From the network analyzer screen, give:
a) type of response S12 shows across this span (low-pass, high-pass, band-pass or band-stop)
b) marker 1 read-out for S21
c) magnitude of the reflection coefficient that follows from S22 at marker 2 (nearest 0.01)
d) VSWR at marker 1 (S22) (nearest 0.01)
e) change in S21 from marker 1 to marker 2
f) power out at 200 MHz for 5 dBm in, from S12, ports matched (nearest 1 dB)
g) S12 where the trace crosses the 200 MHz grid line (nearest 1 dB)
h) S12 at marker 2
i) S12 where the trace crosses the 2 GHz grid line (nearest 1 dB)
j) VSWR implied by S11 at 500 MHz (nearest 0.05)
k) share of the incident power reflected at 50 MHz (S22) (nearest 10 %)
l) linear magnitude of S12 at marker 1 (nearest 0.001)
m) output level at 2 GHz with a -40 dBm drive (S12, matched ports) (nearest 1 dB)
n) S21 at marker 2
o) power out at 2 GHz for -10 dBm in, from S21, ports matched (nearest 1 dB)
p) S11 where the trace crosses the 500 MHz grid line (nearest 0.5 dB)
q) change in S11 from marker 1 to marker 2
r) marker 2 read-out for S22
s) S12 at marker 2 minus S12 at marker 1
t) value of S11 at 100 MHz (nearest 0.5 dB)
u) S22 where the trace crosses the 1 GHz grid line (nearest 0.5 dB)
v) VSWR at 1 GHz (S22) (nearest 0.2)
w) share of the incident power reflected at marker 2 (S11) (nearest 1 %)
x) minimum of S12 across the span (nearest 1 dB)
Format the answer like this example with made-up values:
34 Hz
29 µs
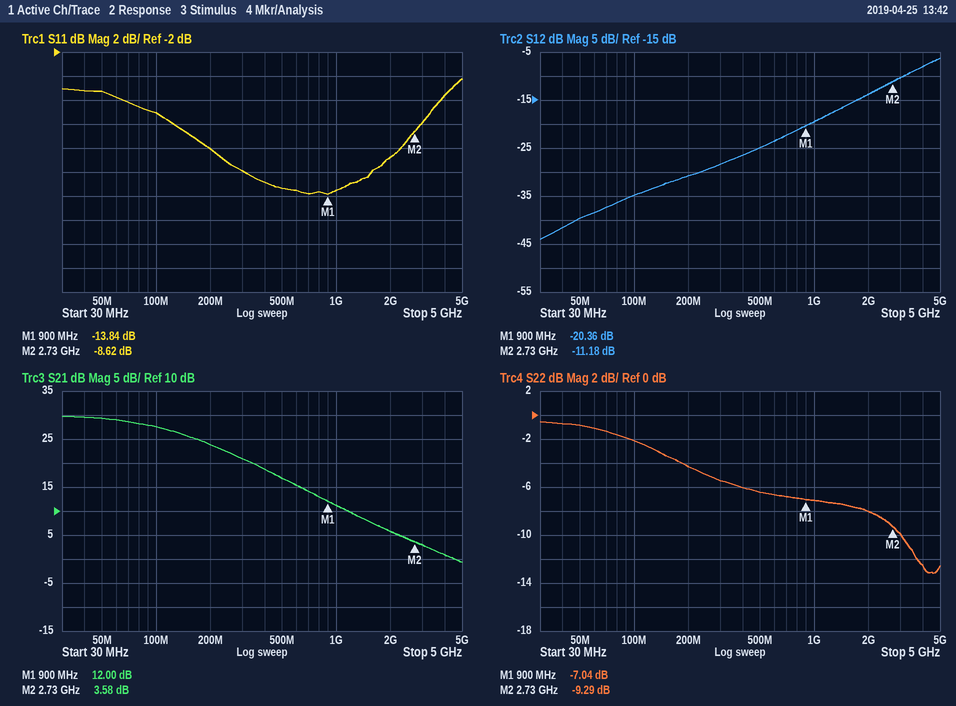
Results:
high-pass
12.00 dB
0.34
2.60
-8.42 dB
-26 dBm
-31 dB
-11.18 dB
-14 dB
1.55
80 %
0.096
-54 dBm
3.58 dB
-4 dBm
-13.5 dB
5.22 dB
-9.29 dB
9.18 dB
-7.0 dB
-7.0 dB
2.6
14 %
-44 dB
